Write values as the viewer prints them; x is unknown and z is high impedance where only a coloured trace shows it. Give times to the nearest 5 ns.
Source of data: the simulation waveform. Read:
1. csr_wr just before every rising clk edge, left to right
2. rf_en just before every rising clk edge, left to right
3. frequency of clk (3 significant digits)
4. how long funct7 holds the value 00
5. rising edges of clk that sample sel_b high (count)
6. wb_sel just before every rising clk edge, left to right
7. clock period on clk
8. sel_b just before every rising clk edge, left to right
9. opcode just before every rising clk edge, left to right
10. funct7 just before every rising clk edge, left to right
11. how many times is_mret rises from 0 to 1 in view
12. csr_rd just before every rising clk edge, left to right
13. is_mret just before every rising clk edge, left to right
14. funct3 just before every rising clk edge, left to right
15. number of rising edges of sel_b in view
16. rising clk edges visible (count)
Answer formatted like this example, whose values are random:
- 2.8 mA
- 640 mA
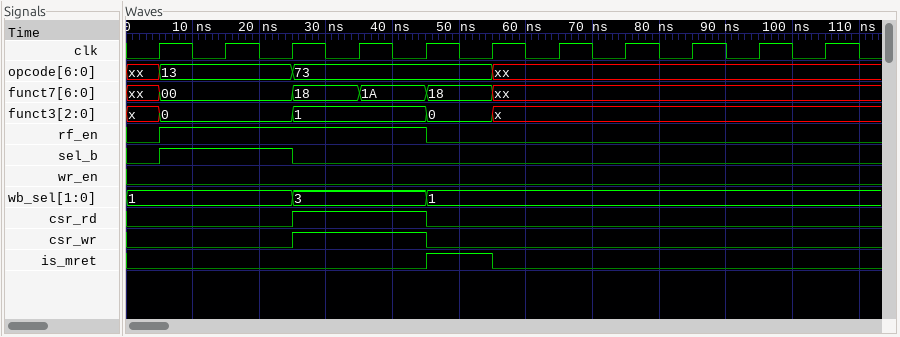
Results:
- 0 0 0 1 1 0 0 0 0 0 0
- 0 1 1 1 1 0 0 0 0 0 0
- 100 MHz
- 20 ns
- 2
- 1, 1, 1, 3, 3, 1, 1, 1, 1, 1, 1
- 10 ns
- 0 1 1 0 0 0 0 0 0 0 0
- xx, 13, 13, 73, 73, 73, xx, xx, xx, xx, xx
- xx, 00, 00, 18, 1A, 18, xx, xx, xx, xx, xx
- 1
- 0 0 0 1 1 0 0 0 0 0 0
- 0 0 0 0 0 1 0 0 0 0 0
- x, 0, 0, 1, 1, 0, x, x, x, x, x
- 1
- 11
